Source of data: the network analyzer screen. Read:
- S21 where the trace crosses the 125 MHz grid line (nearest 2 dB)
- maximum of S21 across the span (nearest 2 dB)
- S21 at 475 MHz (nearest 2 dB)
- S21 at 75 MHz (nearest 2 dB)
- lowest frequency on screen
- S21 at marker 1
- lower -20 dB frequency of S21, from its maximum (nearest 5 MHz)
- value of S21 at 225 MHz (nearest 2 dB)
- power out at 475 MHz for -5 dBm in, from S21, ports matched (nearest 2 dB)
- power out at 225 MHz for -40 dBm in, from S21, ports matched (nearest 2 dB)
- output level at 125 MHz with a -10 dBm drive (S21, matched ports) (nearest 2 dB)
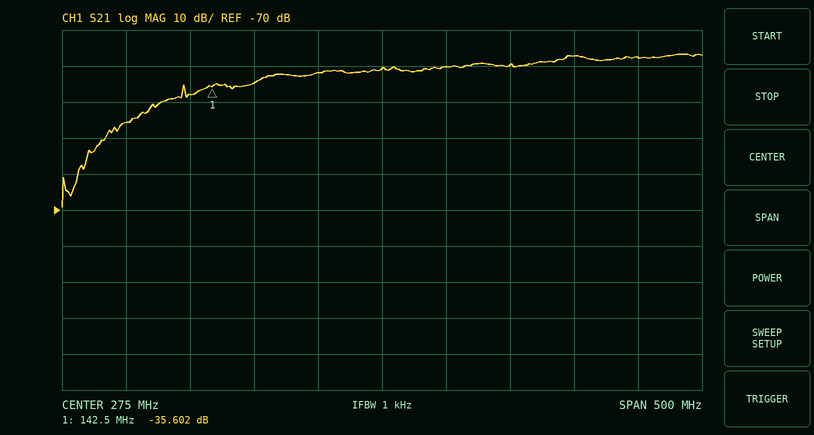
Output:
-38 dB
-26 dB
-28 dB
-46 dB
25 MHz
-35.602 dB
70 MHz
-32 dB
-32 dBm
-72 dBm
-48 dBm
